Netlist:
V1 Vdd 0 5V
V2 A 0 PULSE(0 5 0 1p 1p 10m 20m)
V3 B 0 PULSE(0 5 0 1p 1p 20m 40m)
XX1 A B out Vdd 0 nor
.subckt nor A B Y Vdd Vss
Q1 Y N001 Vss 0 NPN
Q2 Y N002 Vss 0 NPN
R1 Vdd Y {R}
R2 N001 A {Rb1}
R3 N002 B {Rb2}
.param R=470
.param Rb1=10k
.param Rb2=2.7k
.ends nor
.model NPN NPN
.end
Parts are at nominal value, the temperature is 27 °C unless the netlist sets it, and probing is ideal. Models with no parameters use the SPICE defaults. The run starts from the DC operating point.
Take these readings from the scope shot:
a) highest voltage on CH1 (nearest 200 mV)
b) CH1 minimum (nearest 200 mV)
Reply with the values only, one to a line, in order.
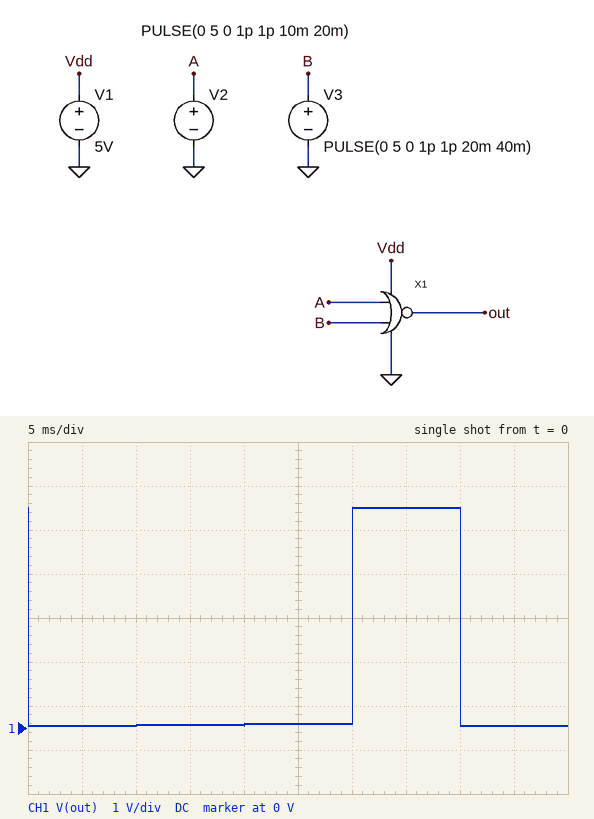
5.0 V
0 V
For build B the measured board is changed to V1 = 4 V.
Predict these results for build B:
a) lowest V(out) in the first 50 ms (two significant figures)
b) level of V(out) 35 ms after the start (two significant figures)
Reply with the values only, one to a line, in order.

49 mV
4.0 V
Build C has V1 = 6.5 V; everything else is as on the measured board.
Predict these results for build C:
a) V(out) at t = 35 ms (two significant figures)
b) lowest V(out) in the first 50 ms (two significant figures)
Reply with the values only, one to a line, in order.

6.5 V
59 mV
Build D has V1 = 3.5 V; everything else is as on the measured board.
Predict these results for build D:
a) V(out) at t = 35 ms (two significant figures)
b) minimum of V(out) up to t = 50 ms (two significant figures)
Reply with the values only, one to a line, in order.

3.5 V
46 mV
